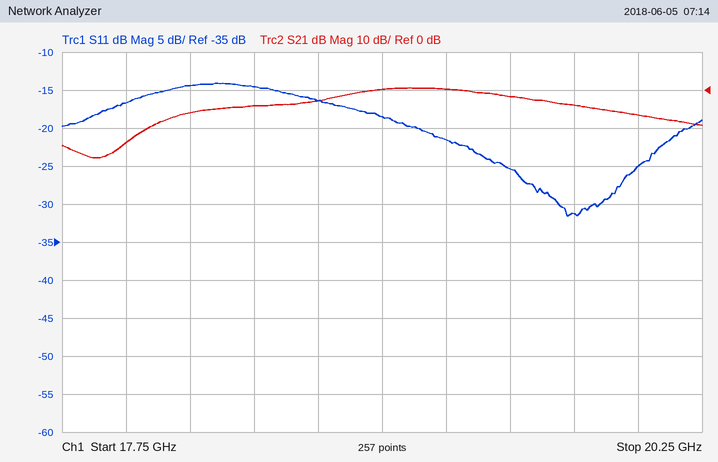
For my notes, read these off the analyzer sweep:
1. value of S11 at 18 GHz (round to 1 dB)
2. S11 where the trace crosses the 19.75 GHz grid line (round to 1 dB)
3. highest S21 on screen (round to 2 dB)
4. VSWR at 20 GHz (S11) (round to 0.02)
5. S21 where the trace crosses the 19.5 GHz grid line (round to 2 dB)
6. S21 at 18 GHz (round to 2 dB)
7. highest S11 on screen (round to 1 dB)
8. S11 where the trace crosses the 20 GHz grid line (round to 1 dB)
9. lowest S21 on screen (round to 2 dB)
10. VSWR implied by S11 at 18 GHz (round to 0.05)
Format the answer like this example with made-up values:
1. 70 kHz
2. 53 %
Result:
1. -17 dB
2. -31 dB
3. 0 dB
4. 1.12
5. -2 dB
6. -14 dB
7. -14 dB
8. -25 dB
9. -18 dB
10. 1.35
